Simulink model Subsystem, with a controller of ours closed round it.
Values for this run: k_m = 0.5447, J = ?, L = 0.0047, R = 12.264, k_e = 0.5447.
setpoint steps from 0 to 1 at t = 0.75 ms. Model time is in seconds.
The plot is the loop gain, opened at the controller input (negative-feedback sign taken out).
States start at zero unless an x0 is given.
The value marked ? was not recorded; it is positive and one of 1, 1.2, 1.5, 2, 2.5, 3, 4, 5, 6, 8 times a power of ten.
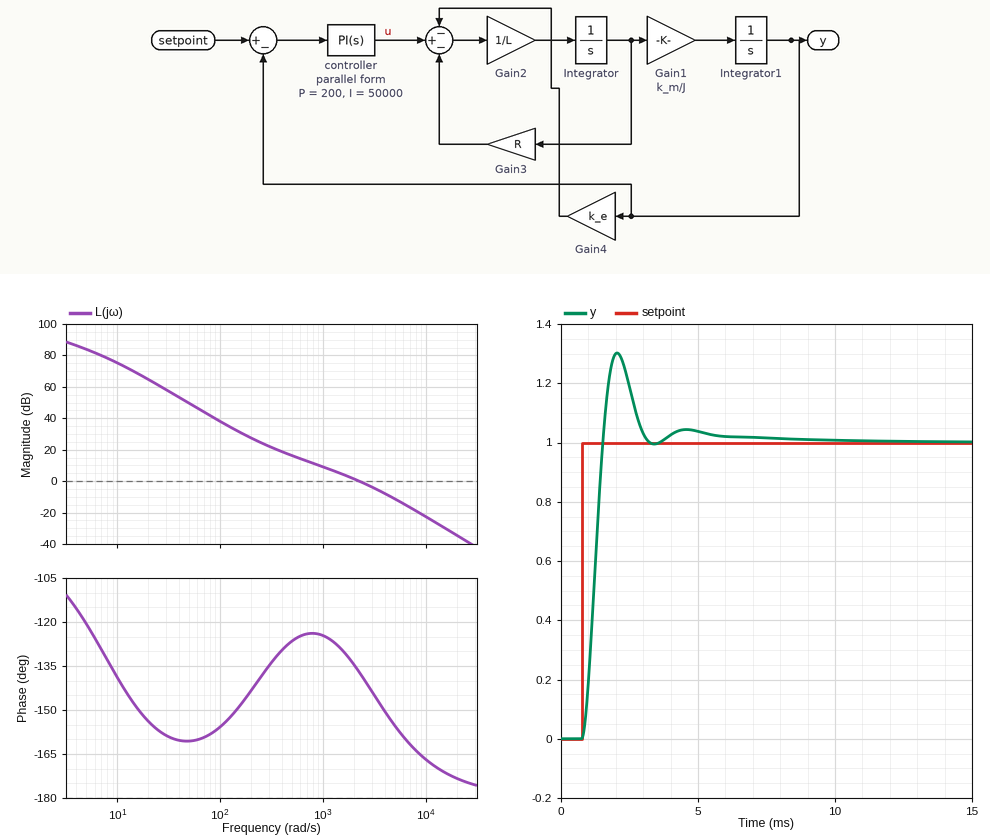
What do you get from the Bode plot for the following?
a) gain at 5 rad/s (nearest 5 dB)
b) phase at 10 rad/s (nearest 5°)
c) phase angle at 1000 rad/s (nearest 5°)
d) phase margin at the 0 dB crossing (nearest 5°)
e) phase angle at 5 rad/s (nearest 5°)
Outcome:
85 dB
-140°
-125°
45°
-120°
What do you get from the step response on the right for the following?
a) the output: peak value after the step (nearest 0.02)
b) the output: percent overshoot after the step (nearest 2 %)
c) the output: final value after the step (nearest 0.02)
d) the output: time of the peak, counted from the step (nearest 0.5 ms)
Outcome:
1.30
30 %
1.00
1.5 ms
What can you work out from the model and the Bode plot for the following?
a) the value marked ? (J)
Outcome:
0.003
